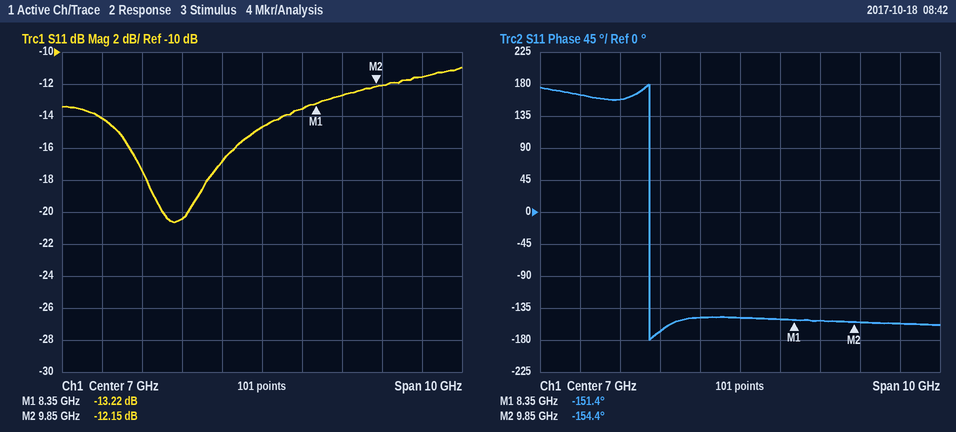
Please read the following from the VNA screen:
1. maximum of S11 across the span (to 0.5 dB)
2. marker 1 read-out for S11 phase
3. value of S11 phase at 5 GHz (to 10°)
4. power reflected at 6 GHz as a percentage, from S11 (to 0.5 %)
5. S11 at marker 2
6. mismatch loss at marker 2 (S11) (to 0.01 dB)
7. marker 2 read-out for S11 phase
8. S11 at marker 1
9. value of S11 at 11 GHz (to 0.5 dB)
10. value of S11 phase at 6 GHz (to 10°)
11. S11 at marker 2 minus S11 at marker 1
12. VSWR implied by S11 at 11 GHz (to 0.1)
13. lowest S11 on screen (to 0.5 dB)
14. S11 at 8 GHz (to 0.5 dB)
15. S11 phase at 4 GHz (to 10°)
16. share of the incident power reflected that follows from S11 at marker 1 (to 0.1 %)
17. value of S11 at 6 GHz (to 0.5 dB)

-11.0 dB
-151.4°
-170°
2.0 %
-12.15 dB
0.27 dB
-154.4°
-13.22 dB
-11.5 dB
-150°
1.07 dB
1.7
-20.5 dB
-13.5 dB
160°
4.8 %
-17.0 dB
